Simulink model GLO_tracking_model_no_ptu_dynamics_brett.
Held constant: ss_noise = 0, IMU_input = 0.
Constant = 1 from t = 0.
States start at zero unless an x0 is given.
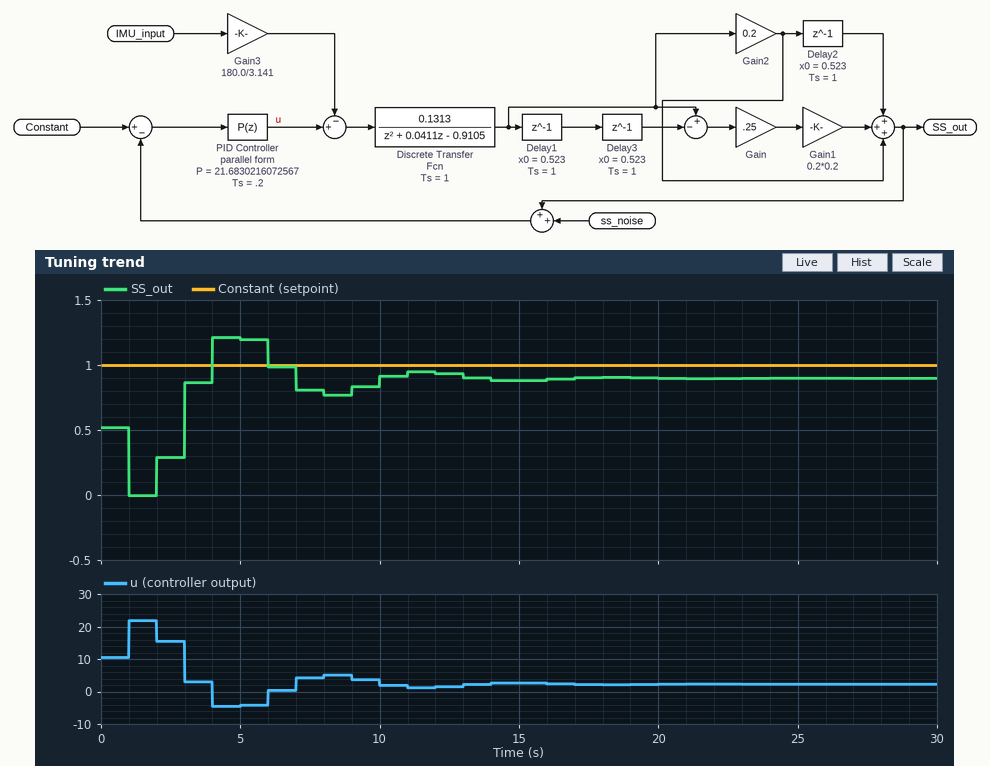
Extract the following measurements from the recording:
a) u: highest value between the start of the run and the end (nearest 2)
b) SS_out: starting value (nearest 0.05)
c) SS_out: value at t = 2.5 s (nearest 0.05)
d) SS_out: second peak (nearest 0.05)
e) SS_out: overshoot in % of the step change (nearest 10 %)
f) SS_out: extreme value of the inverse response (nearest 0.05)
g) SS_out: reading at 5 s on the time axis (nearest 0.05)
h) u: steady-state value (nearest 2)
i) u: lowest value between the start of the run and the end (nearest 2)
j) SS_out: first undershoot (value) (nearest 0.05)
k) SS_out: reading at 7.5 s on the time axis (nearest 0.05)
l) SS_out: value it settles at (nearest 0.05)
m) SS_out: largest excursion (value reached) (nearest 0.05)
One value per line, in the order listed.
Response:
22
0.50
0.30
0.95
80 %
0.00
1.20
2
-4
0.75
0.80
0.90
1.20
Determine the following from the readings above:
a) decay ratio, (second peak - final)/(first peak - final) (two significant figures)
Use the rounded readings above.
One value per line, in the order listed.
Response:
0.17
